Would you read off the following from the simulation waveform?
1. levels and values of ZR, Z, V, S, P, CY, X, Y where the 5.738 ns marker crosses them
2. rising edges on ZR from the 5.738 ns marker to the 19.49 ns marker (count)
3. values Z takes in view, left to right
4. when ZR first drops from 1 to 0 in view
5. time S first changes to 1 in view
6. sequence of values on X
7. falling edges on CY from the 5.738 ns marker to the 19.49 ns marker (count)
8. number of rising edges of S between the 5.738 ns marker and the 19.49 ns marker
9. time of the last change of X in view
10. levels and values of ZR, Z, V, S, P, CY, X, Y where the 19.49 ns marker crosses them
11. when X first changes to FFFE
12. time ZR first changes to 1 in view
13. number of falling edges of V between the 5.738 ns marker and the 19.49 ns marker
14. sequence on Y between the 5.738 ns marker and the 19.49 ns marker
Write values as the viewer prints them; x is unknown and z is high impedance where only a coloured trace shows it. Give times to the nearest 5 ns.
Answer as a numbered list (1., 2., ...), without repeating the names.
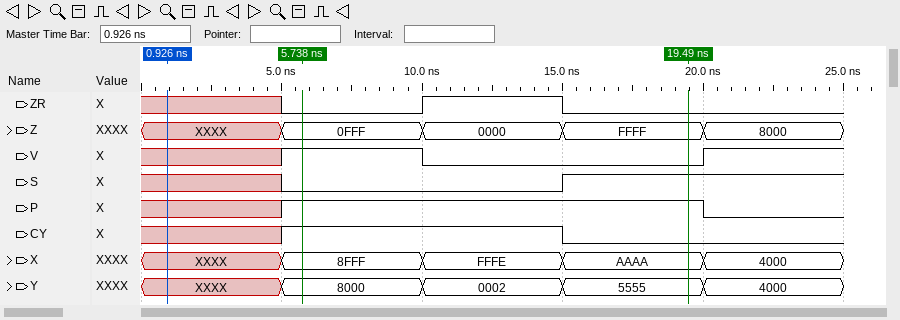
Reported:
1. ZR=0, Z=0FFF, V=1, S=0, P=1, CY=1, X=8FFF, Y=8000
2. 1
3. XXXX, 0FFF, 0000, FFFF, 8000
4. 15 ns
5. 15 ns
6. XXXX, 8FFF, FFFE, AAAA, 4000
7. 1
8. 1
9. 20 ns
10. ZR=0, Z=FFFF, V=0, S=1, P=1, CY=0, X=AAAA, Y=5555
11. 10 ns
12. 10 ns
13. 1
14. 8000, 0002, 5555
